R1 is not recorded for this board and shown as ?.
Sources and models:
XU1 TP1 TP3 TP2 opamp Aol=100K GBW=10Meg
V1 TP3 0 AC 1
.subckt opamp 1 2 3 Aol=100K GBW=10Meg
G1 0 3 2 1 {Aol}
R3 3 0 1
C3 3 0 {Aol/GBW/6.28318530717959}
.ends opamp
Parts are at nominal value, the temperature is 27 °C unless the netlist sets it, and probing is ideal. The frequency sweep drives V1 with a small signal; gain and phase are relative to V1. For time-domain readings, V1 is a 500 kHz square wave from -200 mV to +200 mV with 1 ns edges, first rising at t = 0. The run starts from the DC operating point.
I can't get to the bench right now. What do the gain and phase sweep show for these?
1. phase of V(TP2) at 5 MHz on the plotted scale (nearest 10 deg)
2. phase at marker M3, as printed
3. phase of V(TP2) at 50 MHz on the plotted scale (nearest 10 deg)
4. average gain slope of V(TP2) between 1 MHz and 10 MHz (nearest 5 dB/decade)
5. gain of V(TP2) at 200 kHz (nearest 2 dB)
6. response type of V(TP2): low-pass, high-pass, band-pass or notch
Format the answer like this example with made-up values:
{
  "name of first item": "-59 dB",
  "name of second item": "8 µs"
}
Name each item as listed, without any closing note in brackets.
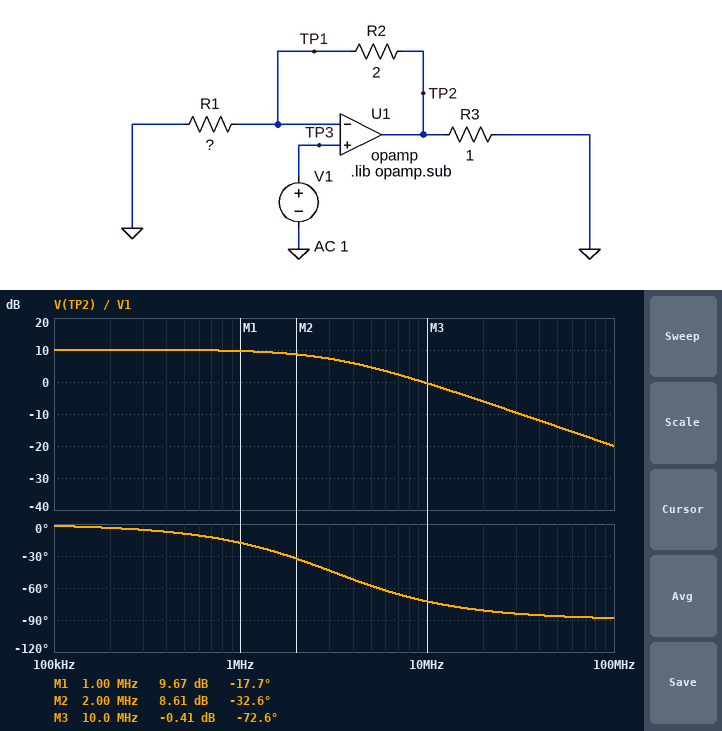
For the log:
{
  "phase of V(TP2) at 5 MHz on the plotted scale": "-60 deg",
  "phase at marker M3, as printed": "-72.6 deg",
  "phase of V(TP2) at 50 MHz on the plotted scale": "-90 deg",
  "average gain slope of V(TP2) between 1 MHz and 10 MHz": "-10 dB/decade",
  "gain of V(TP2) at 200 kHz": "10 dB",
  "response type of V(TP2): low-pass, high-pass, band-pass or notch": "low-pass"
}
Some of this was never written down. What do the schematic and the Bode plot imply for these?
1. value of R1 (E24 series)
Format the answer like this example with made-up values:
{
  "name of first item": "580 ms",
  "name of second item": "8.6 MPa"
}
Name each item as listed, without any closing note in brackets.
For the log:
{
  "value of R1": "0.91 Ω"
}
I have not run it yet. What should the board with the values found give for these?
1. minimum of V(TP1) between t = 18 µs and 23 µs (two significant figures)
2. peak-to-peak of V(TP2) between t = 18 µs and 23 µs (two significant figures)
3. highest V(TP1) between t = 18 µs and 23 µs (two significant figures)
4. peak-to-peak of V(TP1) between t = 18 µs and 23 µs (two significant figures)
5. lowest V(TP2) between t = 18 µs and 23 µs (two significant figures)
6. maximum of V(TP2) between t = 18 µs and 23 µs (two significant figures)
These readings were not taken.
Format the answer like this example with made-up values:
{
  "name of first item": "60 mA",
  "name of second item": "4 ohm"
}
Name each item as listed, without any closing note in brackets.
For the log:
{
  "minimum of V(TP1) between t = 18 µs and 23 µs": "-200 mV",
  "peak-to-peak of V(TP2) between t = 18 µs and 23 µs": "1.3 V",
  "highest V(TP1) between t = 18 µs and 23 µs": "200 mV",
  "peak-to-peak of V(TP1) between t = 18 µs and 23 µs": "400 mV",
  "lowest V(TP2) between t = 18 µs and 23 µs": "-640 mV",
  "maximum of V(TP2) between t = 18 µs and 23 µs": "640 mV"
}
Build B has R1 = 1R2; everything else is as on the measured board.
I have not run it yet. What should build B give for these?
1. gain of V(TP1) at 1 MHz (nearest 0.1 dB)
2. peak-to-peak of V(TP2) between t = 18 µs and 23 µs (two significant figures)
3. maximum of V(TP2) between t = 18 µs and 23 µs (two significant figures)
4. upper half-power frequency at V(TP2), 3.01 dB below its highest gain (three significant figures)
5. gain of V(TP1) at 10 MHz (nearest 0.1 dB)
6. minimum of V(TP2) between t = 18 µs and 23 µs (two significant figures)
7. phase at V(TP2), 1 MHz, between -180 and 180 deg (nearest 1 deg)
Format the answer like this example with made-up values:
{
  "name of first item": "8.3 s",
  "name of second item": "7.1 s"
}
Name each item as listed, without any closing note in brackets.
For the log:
{
  "gain of V(TP1) at 1 MHz": "-0.3 dB",
  "peak-to-peak of V(TP2) between t = 18 µs and 23 µs": "1.1 V",
  "maximum of V(TP2) between t = 18 µs and 23 µs": "530 mV",
  "upper half-power frequency at V(TP2), 3.01 dB below its highest gain": "3.75 MHz",
  "gain of V(TP1) at 10 MHz": "-9.1 dB",
  "minimum of V(TP2) between t = 18 µs and 23 µs": "-530 mV",
  "phase at V(TP2), 1 MHz, between -180 and 180 deg": "-15 deg"
}
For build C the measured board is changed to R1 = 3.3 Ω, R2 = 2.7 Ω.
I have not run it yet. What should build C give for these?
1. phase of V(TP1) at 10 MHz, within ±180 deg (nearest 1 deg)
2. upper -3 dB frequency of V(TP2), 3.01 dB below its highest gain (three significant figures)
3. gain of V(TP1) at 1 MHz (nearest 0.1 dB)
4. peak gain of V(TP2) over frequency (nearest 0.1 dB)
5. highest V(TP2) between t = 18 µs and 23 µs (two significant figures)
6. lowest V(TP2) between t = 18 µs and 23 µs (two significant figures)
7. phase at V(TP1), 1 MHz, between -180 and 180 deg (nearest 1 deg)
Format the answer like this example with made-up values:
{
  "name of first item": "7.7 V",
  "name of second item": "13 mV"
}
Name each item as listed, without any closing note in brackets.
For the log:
{
  "phase of V(TP1) at 10 MHz, within ±180 deg": "-61 deg",
  "upper -3 dB frequency of V(TP2), 3.01 dB below its highest gain": "5.50 MHz",
  "gain of V(TP1) at 1 MHz": "-0.1 dB",
  "peak gain of V(TP2) over frequency": "5.2 dB",
  "highest V(TP2) between t = 18 µs and 23 µs": "360 mV",
  "lowest V(TP2) between t = 18 µs and 23 µs": "-360 mV",
  "phase at V(TP1), 1 MHz, between -180 and 180 deg": "-10 deg"
}
